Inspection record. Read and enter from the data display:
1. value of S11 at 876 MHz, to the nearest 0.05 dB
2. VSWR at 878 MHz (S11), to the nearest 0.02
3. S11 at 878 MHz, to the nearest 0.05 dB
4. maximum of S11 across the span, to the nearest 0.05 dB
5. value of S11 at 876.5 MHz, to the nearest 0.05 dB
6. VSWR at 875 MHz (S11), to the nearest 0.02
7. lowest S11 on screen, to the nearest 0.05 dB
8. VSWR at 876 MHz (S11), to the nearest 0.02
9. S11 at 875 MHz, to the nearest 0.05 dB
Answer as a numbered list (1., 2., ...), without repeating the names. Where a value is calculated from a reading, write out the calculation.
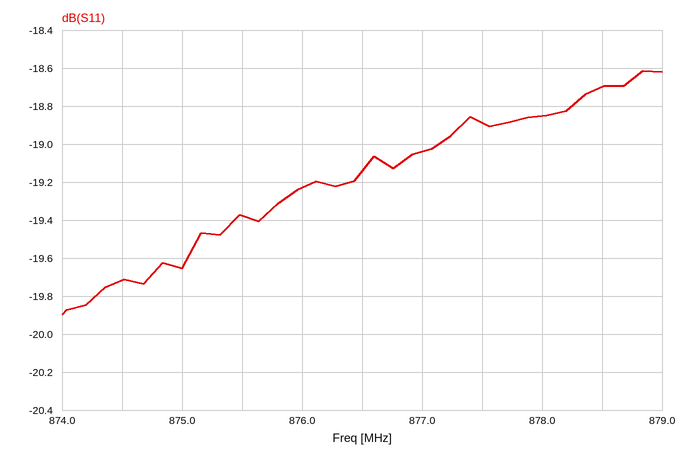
1. -19.25 dB
2. |Γ| = 10^(-18.85/20) = 0.1142; VSWR = (1 + 0.1142)/(1 − 0.1142) ≈ 1.26
3. -18.85 dB
4. -18.60 dB
5. -19.15 dB
6. |Γ| = 10^(-19.65/20) = 0.1041; VSWR = (1 + 0.1041)/(1 − 0.1041) ≈ 1.23, so 1.24 to the nearest 0.02
7. -19.90 dB
8. |Γ| = 10^(-19.25/20) = 0.1090; VSWR = (1 + 0.1090)/(1 − 0.1090) ≈ 1.24
9. -19.65 dB
